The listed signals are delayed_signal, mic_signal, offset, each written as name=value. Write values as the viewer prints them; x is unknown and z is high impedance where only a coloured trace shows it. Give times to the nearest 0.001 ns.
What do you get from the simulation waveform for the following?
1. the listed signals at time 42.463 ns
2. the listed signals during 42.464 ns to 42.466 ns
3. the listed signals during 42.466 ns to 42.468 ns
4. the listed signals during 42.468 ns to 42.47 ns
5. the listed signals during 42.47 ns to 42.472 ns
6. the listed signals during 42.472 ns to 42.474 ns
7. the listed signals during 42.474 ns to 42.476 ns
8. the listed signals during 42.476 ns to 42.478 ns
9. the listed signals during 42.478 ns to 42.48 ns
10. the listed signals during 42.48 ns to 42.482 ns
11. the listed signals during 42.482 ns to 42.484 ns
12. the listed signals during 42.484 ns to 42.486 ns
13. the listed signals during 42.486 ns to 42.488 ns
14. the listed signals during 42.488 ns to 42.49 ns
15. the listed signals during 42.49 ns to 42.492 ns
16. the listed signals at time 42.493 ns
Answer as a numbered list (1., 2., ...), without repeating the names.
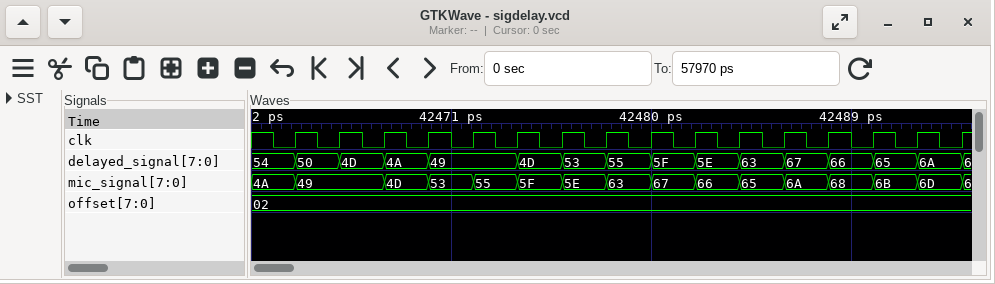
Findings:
1. delayed_signal=54, mic_signal=4A, offset=02
2. delayed_signal=50, mic_signal=49, offset=02
3. delayed_signal=4D, mic_signal=49, offset=02
4. delayed_signal=4A, mic_signal=4D, offset=02
5. delayed_signal=49, mic_signal=53, offset=02
6. delayed_signal=49, mic_signal=55, offset=02
7. delayed_signal=4D, mic_signal=5F, offset=02
8. delayed_signal=53, mic_signal=5E, offset=02
9. delayed_signal=55, mic_signal=63, offset=02
10. delayed_signal=5F, mic_signal=67, offset=02
11. delayed_signal=5E, mic_signal=66, offset=02
12. delayed_signal=63, mic_signal=65, offset=02
13. delayed_signal=67, mic_signal=6A, offset=02
14. delayed_signal=66, mic_signal=68, offset=02
15. delayed_signal=65, mic_signal=6B, offset=02
16. delayed_signal=6A, mic_signal=6D, offset=02
